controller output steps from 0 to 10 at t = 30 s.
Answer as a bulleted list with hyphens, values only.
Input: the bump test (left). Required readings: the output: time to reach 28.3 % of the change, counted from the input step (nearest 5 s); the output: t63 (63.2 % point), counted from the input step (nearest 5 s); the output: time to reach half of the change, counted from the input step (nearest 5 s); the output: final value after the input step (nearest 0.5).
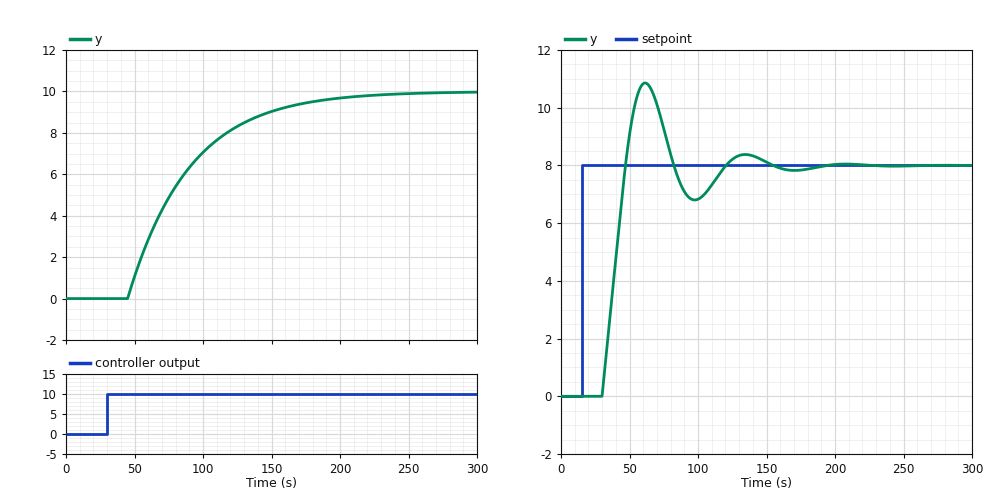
- 30 s
- 60 s
- 45 s
- 10.0
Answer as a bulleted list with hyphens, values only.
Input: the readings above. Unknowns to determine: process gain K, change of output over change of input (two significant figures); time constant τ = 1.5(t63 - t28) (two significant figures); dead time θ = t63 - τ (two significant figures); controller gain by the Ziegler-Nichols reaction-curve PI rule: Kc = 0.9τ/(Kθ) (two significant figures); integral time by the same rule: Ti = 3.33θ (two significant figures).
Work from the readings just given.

- 1.0
- 45 s
- 15 s
- 2.7
- 50 s
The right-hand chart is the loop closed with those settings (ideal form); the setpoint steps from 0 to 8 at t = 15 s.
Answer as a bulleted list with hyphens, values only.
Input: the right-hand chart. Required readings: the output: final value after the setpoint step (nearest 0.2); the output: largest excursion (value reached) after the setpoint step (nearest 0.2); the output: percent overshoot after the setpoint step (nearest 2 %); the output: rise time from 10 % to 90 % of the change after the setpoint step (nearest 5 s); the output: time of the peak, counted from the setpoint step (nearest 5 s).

- 8.0
- 10.8
- 36 %
- 15 s
- 45 s
